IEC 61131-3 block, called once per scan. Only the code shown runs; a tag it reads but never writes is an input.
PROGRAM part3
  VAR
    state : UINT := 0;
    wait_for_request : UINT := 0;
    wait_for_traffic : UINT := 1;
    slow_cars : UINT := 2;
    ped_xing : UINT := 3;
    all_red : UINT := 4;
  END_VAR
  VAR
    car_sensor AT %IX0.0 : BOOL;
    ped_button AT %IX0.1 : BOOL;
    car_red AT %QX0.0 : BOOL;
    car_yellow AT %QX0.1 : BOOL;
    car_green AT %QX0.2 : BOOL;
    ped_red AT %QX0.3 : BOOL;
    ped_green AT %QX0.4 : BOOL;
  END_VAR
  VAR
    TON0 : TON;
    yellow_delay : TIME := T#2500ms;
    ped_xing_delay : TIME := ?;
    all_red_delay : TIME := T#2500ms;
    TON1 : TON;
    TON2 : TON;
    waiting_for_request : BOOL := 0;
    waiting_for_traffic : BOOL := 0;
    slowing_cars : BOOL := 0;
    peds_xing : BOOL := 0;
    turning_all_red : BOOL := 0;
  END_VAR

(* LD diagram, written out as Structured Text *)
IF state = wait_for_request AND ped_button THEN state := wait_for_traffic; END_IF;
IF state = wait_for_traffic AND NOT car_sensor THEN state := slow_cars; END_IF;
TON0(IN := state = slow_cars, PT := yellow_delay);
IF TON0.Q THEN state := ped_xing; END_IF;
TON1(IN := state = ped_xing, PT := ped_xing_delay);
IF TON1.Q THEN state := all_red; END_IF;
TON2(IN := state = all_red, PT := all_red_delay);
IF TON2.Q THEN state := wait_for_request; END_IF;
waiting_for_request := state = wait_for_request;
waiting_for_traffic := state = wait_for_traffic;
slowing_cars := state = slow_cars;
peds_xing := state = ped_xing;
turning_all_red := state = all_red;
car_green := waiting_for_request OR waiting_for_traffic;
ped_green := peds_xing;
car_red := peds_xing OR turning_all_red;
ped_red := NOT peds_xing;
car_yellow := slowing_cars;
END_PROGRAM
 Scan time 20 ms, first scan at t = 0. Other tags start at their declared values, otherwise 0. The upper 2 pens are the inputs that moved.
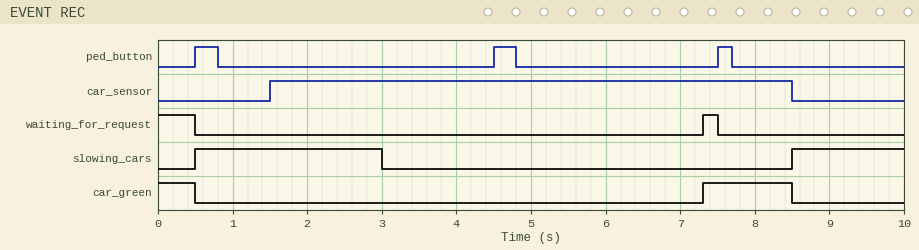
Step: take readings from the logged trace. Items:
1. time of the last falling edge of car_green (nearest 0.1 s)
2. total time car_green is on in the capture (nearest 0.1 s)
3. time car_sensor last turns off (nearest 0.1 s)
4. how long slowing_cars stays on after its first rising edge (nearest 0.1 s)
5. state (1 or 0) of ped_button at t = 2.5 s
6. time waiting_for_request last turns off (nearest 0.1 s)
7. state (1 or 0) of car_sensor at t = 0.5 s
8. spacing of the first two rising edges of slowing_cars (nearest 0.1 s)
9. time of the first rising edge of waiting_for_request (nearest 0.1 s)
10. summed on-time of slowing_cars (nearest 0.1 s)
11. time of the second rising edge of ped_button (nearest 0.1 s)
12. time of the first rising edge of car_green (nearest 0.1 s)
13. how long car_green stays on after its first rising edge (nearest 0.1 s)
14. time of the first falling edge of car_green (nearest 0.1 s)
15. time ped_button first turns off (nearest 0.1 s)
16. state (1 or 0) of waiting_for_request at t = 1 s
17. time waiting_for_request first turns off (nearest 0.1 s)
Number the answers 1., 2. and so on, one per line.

1. 8.5 s
2. 1.7 s
3. 8.5 s
4. 2.5 s
5. 0
6. 7.5 s
7. 0
8. 8.0 s
9. 7.3 s
10. 4.0 s
11. 4.5 s
12. 7.3 s
13. 1.2 s
14. 0.5 s
15. 0.8 s
16. 0
17. 0.5 s
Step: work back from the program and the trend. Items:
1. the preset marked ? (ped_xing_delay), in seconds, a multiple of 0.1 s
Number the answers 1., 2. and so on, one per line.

1. 1.8 s
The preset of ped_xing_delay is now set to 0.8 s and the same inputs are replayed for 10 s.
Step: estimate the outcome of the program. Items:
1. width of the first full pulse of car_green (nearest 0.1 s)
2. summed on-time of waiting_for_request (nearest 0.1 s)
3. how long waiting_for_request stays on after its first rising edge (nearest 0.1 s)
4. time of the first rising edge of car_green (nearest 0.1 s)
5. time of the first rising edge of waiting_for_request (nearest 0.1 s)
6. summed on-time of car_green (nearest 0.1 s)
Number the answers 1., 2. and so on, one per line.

1. 2.2 s
2. 1.7 s
3. 1.2 s
4. 6.3 s
5. 6.3 s
6. 2.7 s
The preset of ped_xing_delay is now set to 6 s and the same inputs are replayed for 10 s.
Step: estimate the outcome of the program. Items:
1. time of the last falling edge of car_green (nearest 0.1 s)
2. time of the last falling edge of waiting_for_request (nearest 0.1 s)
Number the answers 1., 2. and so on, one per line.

1. 0.5 s
2. 0.5 s
